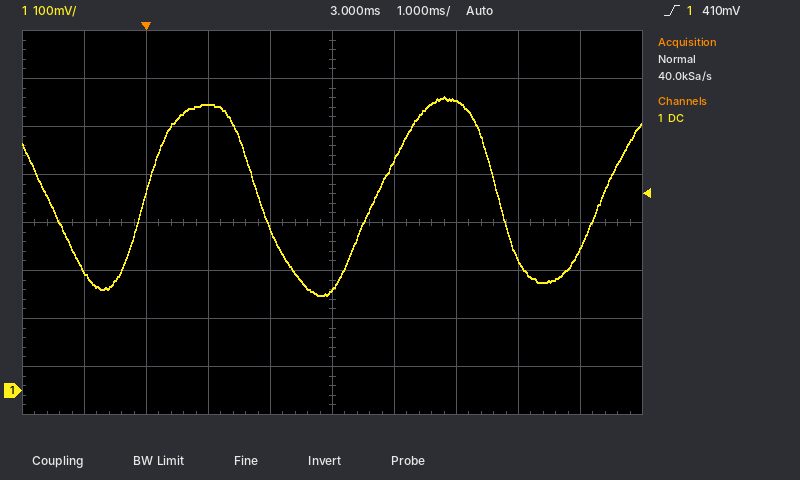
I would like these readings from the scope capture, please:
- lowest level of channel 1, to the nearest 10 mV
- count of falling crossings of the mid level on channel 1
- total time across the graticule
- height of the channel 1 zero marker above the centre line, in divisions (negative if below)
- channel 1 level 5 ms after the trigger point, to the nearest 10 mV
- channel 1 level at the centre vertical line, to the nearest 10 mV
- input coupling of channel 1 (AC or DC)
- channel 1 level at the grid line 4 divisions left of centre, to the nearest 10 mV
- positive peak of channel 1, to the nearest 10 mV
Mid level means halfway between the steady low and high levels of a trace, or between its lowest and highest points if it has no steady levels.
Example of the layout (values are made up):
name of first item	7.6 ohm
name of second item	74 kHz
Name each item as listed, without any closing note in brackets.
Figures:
lowest level of channel 1, to the nearest 10 mV	200 mV
count of falling crossings of the mid level on channel 1	3
total time across the graticule	10 ms
height of the channel 1 zero marker above the centre line, in divisions	-3.5 div
channel 1 level 5 ms after the trigger point, to the nearest 10 mV	600 mV
channel 1 level at the centre vertical line, to the nearest 10 mV	210 mV
input coupling of channel 1	DC
channel 1 level at the grid line 4 divisions left of centre, to the nearest 10 mV	250 mV
positive peak of channel 1, to the nearest 10 mV	610 mV
